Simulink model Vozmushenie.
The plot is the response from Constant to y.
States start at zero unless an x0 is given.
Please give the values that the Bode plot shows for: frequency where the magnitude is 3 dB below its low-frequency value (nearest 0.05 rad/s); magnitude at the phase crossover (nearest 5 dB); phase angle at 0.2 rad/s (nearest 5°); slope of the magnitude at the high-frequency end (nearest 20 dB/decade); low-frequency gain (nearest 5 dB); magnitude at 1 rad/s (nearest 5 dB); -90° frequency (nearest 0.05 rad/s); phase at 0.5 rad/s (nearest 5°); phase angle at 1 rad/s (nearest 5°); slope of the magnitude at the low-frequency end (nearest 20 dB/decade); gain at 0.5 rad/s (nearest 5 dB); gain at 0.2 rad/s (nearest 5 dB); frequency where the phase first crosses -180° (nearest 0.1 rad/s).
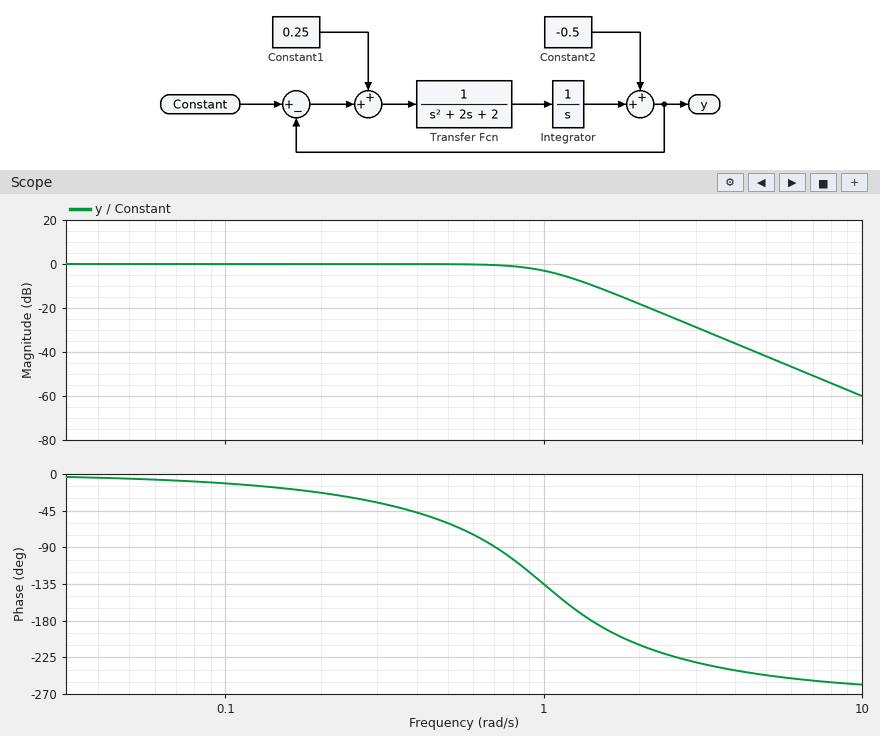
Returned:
1.00 rad/s
-10 dB
-25°
-60 dB/decade
0 dB
-5 dB
0.70 rad/s
-60°
-135°
0 dB/decade
0 dB
0 dB
1.4 rad/s
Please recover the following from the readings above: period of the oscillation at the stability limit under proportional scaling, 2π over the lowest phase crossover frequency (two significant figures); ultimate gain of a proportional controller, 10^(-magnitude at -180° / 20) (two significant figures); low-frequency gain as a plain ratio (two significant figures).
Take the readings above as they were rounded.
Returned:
4.5 s
3.2
1.0
